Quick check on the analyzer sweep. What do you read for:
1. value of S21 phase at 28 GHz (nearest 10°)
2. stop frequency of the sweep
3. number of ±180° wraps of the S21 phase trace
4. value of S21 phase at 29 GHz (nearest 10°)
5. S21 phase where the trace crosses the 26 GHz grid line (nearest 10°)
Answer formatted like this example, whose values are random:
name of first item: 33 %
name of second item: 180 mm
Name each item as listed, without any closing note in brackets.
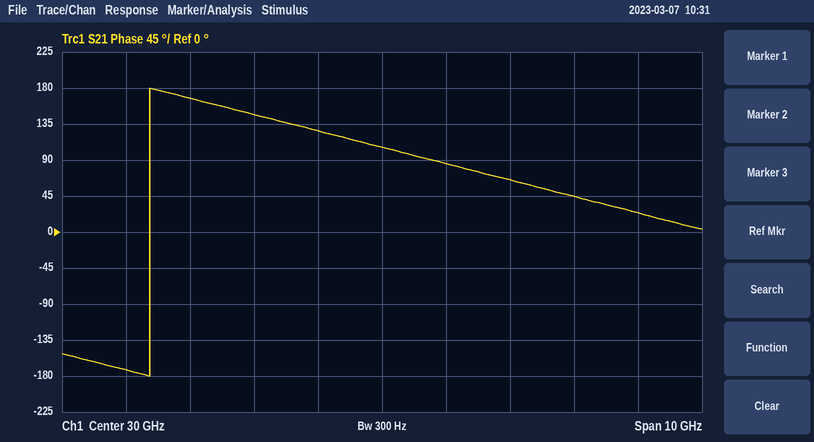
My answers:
value of S21 phase at 28 GHz: 150°
stop frequency of the sweep: 35 GHz
number of ±180° wraps of the S21 phase trace: 1
value of S21 phase at 29 GHz: 130°
S21 phase where the trace crosses the 26 GHz grid line: -170°
